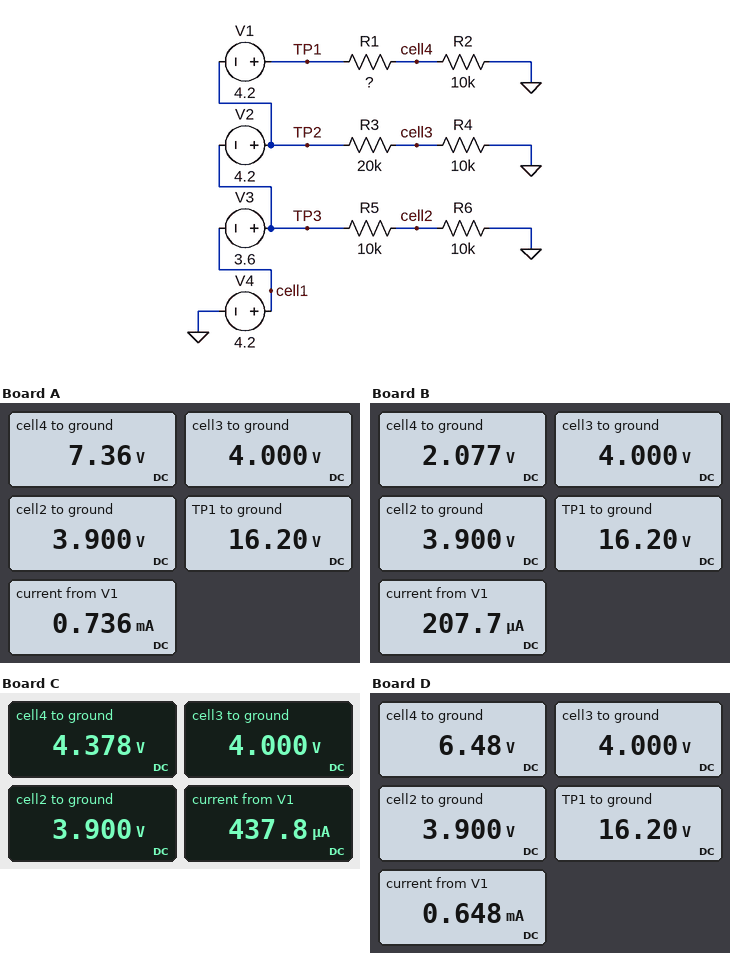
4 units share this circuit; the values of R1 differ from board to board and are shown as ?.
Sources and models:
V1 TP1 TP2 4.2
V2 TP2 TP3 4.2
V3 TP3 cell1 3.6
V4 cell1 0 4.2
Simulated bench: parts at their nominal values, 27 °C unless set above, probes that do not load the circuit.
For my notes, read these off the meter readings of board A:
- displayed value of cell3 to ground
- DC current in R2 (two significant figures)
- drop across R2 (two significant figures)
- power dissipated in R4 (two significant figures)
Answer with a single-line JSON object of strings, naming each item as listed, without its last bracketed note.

{"displayed value of cell3 to ground": "4.000 V", "DC current in R2": "740 µA", "drop across R2": "7.4 V", "power dissipated in R4": "1.6 mW"}
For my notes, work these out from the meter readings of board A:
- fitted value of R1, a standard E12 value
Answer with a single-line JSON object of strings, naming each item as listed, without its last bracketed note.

{"fitted value of R1, a standard E12 value": "12 kΩ"}
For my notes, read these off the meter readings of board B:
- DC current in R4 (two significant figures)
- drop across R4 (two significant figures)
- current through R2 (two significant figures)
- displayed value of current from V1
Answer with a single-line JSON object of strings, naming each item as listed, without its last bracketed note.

{"DC current in R4": "400 µA", "drop across R4": "4.0 V", "current through R2": "210 µA", "displayed value of current from V1": "207.7 µA"}
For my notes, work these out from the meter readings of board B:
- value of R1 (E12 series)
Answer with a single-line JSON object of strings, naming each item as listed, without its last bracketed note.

{"value of R1": "68 kΩ"}
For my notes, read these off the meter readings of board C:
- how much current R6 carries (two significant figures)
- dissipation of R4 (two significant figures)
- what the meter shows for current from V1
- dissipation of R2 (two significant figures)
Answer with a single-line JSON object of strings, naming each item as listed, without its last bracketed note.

{"how much current R6 carries": "390 µA", "dissipation of R4": "1.6 mW", "what the meter shows for current from V1": "437.8 µA", "dissipation of R2": "1.9 mW"}
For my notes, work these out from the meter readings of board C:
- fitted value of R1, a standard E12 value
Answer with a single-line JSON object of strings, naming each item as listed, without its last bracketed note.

{"fitted value of R1, a standard E12 value": "27 kΩ"}
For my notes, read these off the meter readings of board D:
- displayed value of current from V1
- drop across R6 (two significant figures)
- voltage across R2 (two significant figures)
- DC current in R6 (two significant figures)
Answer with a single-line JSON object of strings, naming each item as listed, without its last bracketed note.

{"displayed value of current from V1": "0.648 mA", "drop across R6": "3.9 V", "voltage across R2": "6.5 V", "DC current in R6": "390 µA"}
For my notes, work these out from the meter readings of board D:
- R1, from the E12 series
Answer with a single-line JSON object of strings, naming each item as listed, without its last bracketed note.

{"R1, from the E12 series": "15 kΩ"}
